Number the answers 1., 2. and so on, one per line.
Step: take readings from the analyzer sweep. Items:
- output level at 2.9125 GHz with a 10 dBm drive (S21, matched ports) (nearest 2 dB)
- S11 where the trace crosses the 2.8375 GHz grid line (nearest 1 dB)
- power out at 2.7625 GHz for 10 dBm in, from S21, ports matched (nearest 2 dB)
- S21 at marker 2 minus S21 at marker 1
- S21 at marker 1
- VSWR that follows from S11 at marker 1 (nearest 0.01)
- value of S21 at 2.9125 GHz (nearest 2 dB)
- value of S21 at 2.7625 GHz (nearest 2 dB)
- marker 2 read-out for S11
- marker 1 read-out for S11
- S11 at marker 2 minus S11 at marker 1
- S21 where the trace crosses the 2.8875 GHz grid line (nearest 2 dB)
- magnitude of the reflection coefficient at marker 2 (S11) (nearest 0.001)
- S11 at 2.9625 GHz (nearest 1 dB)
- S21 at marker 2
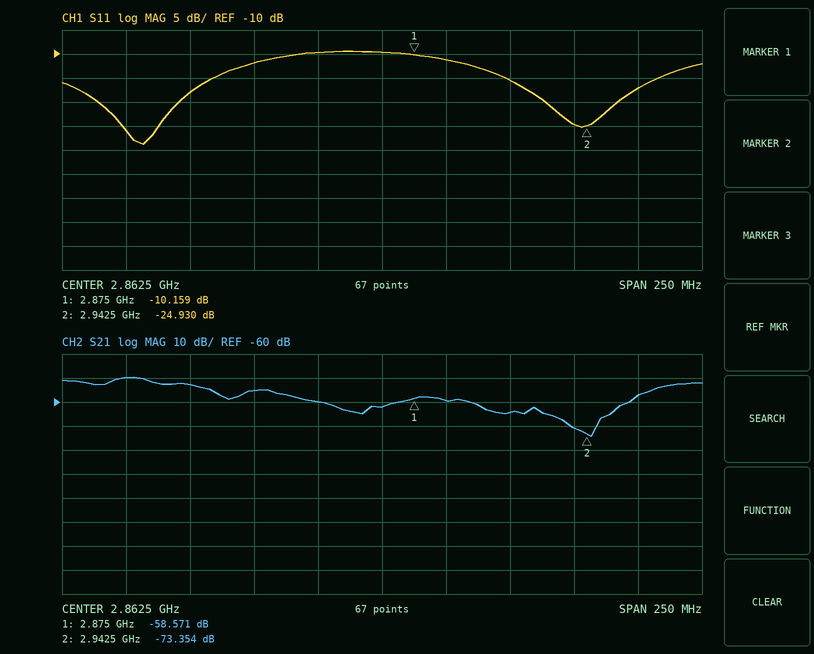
1. -54 dBm
2. -10 dB
3. -40 dBm
4. -14.783 dB
5. -58.571 dB
6. 1.90
7. -64 dB
8. -50 dB
9. -24.930 dB
10. -10.159 dB
11. -14.771 dB
12. -60 dB
13. 0.057
14. -17 dB
15. -73.354 dB
